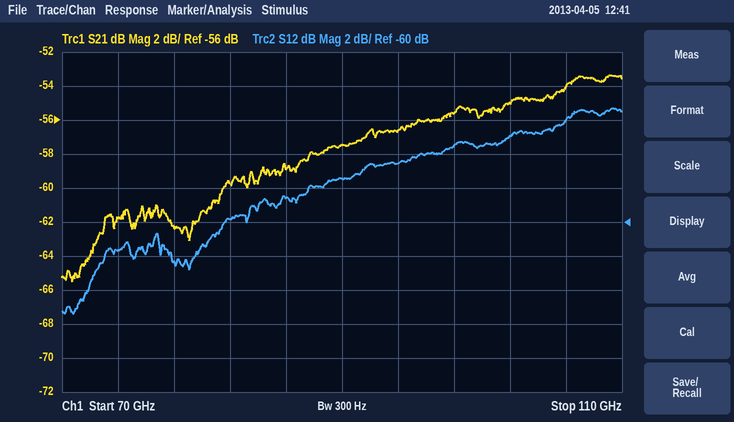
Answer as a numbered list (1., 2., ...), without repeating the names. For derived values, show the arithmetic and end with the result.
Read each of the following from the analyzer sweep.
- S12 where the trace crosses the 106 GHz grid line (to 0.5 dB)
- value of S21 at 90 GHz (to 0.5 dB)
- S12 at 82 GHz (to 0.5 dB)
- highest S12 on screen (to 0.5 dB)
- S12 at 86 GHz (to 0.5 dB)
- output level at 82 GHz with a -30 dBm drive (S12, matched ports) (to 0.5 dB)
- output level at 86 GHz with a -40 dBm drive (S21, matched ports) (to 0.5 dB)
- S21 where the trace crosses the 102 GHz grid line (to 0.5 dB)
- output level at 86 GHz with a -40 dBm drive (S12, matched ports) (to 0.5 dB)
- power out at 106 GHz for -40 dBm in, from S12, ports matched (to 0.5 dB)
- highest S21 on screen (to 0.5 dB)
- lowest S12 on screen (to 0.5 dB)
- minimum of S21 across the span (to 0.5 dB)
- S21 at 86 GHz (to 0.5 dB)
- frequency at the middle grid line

1. -54.0 dB
2. -57.5 dB
3. -60.0 dB
4. -53.5 dB
5. -58.5 dB
6. -30 dBm + (-60.0 dB) = -90.0 dBm
7. -40 dBm + (-59.0 dB) = -99.0 dBm
8. -55.0 dB
9. -40 dBm + (-58.5 dB) = -98.5 dBm
10. -40 dBm + (-54.0 dB) = -94.0 dBm
11. -53.5 dB
12. -65.5 dB
13. -65.5 dB
14. -59.0 dB
15. 90 GHz
